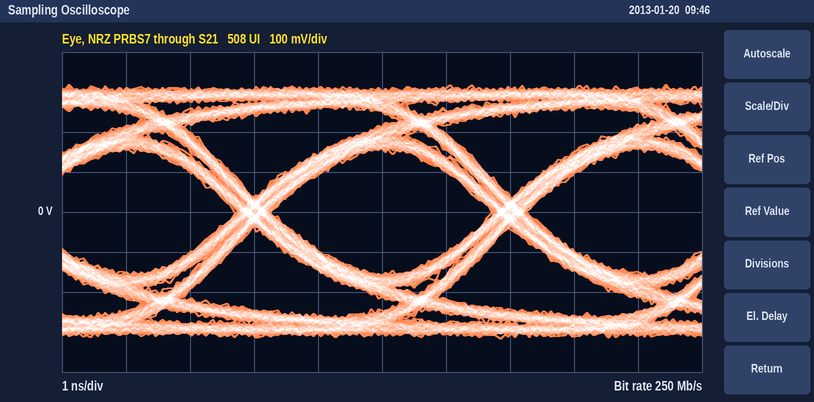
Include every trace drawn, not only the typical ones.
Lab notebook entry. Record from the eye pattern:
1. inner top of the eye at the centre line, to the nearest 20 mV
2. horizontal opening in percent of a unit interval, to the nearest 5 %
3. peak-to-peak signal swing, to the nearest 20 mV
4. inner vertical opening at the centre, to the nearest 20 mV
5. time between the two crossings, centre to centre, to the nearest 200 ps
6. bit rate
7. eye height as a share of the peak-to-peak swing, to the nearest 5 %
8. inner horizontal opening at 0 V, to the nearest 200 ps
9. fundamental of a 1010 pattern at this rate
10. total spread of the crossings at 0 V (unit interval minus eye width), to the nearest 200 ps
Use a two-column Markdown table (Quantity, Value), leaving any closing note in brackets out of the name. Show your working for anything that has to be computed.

| Quantity | Value |
|---|---|
| inner top of the eye at the centre line, to the nearest 20 mV | 160 mV |
| horizontal opening in percent of a unit interval, to the nearest 5 % | 3.4 ns / 4.0 ns ≈ 85 % |
| peak-to-peak signal swing, to the nearest 20 mV | 640 mV |
| inner vertical opening at the centre, to the nearest 20 mV | 320 mV |
| time between the two crossings, centre to centre, to the nearest 200 ps | 4.0 ns |
| bit rate | 250 Mb/s |
| eye height as a share of the peak-to-peak swing, to the nearest 5 % | 320 mV / 640 mV ≈ 50 % |
| inner horizontal opening at 0 V, to the nearest 200 ps | 3.4 ns |
| fundamental of a 1010 pattern at this rate | 125 MHz |
| total spread of the crossings at 0 V (unit interval minus eye width), to the nearest 200 ps | 600 ps |
